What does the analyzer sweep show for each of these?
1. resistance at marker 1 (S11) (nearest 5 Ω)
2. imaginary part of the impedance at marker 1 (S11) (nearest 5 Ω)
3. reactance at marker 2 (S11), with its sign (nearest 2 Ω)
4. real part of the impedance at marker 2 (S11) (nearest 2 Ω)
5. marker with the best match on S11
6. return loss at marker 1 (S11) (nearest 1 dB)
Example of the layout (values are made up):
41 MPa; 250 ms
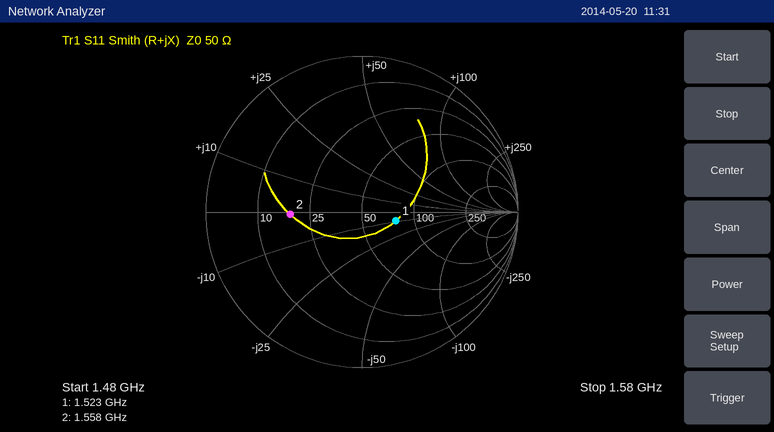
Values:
75 Ω; -10 Ω; 0 Ω; 18 Ω; marker 1; 13 dB
